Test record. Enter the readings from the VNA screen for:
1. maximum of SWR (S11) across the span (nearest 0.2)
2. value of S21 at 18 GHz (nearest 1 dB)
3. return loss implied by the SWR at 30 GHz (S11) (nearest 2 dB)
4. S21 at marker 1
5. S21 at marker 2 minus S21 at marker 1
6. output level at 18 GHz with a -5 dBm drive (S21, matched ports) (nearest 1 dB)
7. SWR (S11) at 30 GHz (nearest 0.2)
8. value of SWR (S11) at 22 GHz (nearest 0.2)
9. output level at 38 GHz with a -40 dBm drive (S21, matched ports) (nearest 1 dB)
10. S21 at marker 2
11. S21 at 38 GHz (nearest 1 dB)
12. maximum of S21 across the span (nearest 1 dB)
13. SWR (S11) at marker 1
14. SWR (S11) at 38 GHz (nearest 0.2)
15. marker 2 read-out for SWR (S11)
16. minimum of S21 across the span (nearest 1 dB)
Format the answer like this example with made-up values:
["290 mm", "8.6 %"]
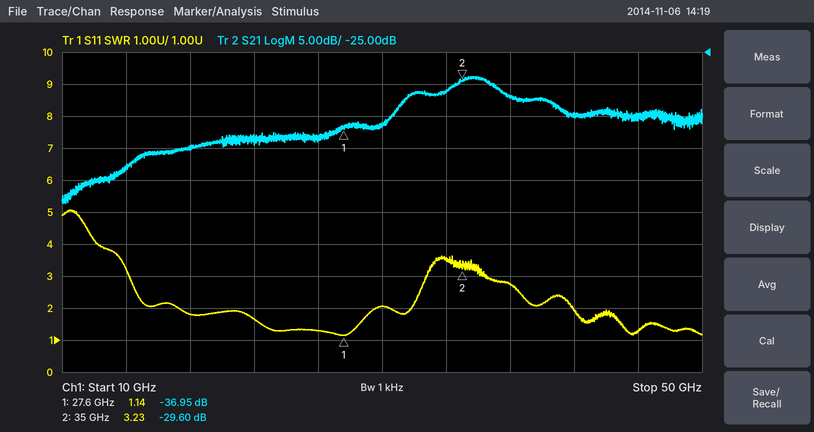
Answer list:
["5.0", "-40 dB", "10 dB", "-36.95 dB", "7.35 dB", "-45 dBm", "2.0", "1.6", "-72 dBm", "-29.60 dB", "-32 dB", "-29 dB", "1.14", "2.8", "3.23", "-49 dB"]
